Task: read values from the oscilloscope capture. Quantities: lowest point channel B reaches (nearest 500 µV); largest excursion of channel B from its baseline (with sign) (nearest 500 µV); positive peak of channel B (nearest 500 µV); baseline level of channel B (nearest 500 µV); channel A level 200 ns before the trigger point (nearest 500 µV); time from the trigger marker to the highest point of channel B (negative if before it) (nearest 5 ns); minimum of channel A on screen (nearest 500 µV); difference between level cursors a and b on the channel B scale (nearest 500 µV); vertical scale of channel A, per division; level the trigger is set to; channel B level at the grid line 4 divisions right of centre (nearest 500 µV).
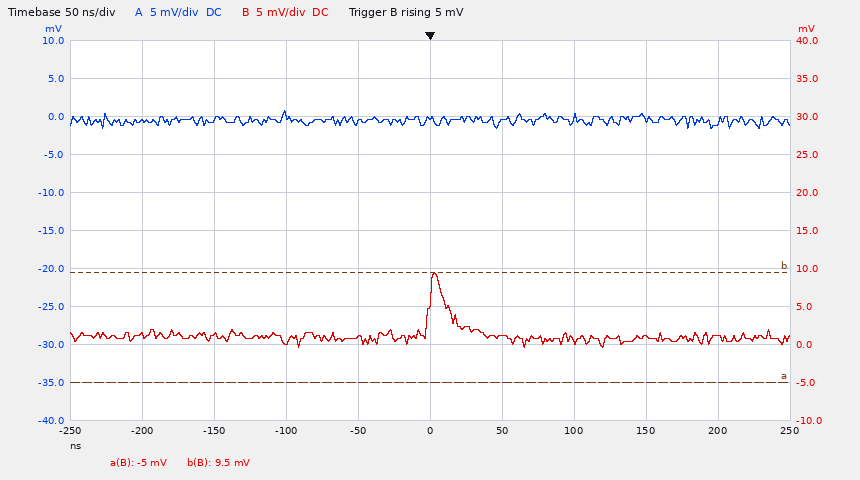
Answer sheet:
-500 µV
+8.5 mV
9.5 mV
1.0 mV
-500 µV
+5 ns
-1.5 mV
14.5 mV
5 mV
5 mV
1.0 mV
